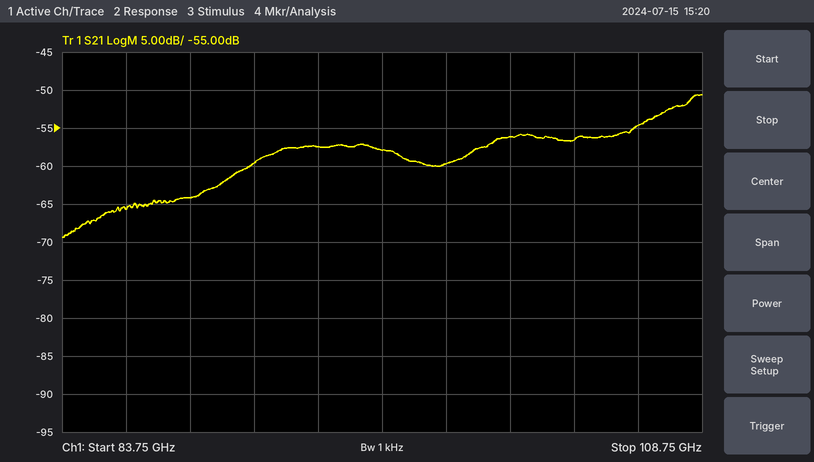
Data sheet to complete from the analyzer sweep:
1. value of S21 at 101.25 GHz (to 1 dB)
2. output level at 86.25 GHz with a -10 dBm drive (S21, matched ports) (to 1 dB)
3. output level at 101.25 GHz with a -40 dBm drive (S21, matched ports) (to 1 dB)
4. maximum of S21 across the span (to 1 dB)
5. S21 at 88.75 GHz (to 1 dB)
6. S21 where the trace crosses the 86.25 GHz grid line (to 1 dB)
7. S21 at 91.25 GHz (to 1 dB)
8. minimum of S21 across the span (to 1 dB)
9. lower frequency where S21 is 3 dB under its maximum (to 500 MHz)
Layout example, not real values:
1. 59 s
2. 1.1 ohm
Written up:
1. -56 dB
2. -76 dBm
3. -96 dBm
4. -51 dB
5. -64 dB
6. -66 dB
7. -60 dB
8. -69 dB
9. 107.0 GHz
